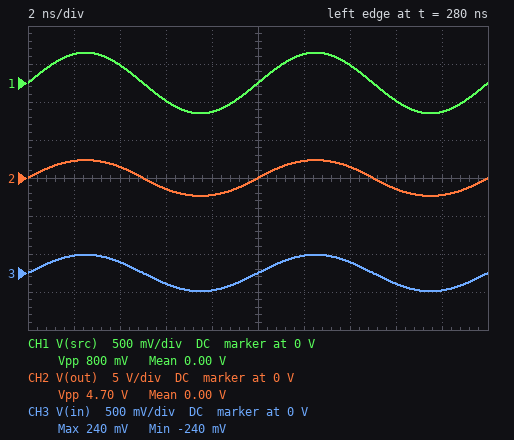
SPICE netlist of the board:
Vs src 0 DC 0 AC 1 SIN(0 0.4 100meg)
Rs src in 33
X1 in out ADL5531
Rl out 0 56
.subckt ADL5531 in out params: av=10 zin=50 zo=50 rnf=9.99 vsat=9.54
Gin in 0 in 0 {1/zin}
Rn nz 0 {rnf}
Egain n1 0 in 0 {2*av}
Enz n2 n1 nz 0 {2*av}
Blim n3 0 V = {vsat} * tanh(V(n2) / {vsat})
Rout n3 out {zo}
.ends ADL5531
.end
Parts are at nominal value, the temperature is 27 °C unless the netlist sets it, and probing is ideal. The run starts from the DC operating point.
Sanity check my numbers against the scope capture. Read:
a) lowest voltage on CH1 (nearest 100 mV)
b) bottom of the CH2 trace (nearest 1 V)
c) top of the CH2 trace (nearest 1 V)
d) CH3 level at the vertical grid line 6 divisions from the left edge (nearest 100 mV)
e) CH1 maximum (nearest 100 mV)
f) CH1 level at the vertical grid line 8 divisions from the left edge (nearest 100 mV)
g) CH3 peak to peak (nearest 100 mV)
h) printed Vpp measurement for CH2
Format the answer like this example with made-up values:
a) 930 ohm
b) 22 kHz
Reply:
a) -400 mV
b) -2 V
c) 2 V
d) 200 mV
e) 400 mV
f) -200 mV
g) 500 mV
h) 4.70 V
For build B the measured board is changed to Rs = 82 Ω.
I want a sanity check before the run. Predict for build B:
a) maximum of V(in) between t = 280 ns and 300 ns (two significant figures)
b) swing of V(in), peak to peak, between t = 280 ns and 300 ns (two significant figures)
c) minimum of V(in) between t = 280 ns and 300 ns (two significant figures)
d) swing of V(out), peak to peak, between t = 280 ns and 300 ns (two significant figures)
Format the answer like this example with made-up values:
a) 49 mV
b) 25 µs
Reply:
a) 150 mV
b) 300 mV
c) -150 mV
d) 3.1 V
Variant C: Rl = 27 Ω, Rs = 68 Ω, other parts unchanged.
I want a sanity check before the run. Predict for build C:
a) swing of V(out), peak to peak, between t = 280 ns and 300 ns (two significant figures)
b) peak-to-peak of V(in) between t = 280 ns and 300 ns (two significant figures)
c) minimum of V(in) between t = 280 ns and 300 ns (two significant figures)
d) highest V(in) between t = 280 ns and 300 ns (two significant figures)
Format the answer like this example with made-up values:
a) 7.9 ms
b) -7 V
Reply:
a) 2.3 V
b) 340 mV
c) -170 mV
d) 170 mV
